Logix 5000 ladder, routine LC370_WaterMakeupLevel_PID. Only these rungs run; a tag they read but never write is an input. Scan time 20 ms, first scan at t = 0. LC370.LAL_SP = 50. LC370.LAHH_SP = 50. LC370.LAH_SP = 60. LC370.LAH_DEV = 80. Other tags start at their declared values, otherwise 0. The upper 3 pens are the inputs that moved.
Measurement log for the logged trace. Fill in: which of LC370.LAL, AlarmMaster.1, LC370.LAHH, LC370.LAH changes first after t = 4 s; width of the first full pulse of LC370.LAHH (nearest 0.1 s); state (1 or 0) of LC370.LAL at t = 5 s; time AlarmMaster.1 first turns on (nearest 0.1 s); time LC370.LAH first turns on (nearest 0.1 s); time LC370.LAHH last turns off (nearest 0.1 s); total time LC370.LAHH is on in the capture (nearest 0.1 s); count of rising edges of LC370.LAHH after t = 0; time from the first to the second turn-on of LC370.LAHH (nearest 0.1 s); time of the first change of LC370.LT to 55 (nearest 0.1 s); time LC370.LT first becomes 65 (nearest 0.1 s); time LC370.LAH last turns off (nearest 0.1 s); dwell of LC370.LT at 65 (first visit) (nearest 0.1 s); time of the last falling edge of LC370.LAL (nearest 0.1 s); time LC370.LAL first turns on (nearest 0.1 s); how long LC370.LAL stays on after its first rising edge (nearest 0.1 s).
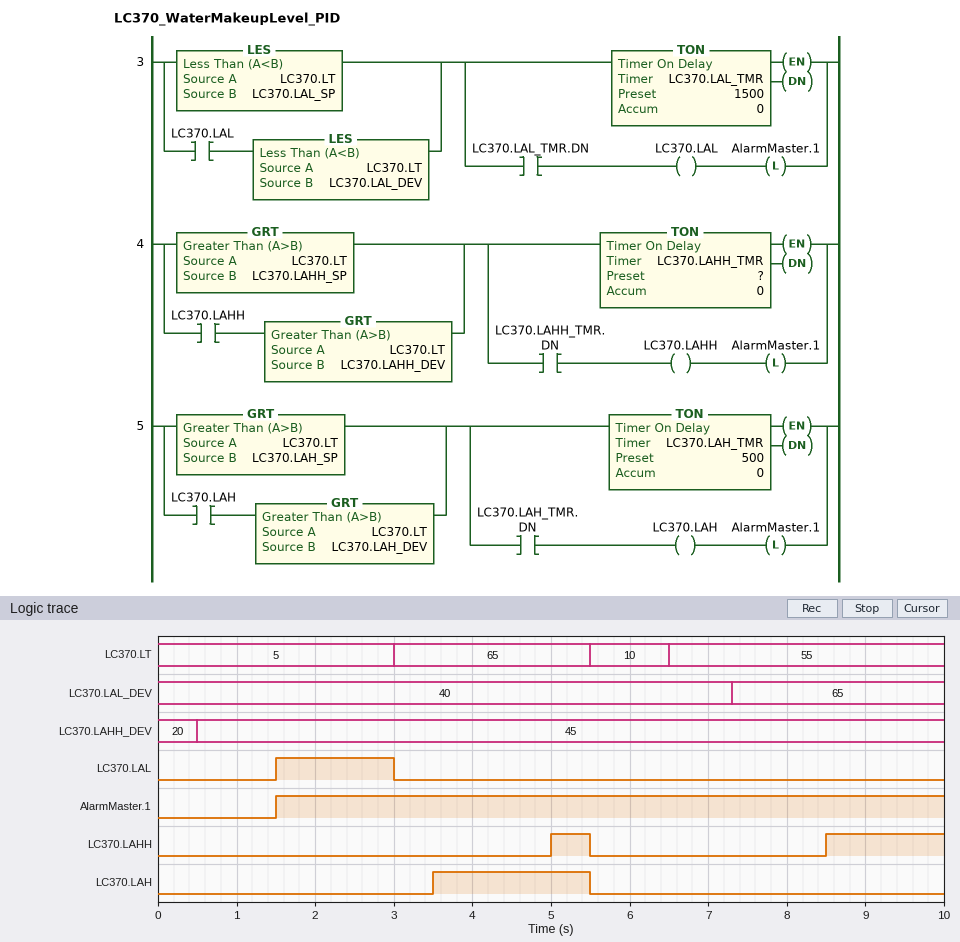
LC370.LAHH
0.5 s
0
1.5 s
3.5 s
5.5 s
2.0 s
2
3.5 s
6.5 s
3.0 s
5.5 s
2.5 s
3.0 s
1.5 s
1.5 s
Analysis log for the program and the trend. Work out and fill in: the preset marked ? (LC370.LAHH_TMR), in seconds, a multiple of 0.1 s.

2.0 s
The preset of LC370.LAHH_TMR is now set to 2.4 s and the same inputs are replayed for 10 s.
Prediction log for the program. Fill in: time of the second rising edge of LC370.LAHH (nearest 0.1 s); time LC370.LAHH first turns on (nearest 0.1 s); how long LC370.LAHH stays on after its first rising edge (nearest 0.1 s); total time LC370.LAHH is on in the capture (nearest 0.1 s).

8.9 s
5.4 s
0.1 s
1.2 s
